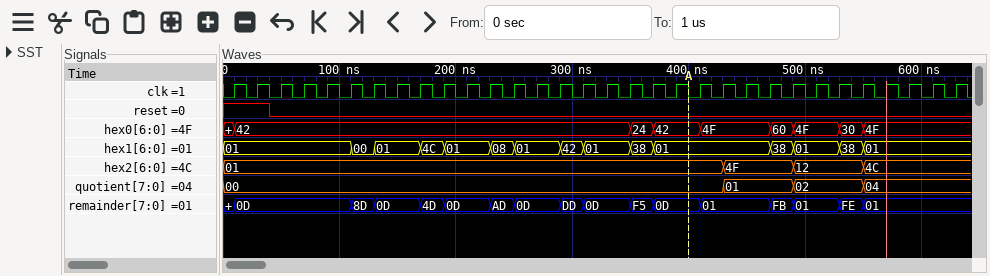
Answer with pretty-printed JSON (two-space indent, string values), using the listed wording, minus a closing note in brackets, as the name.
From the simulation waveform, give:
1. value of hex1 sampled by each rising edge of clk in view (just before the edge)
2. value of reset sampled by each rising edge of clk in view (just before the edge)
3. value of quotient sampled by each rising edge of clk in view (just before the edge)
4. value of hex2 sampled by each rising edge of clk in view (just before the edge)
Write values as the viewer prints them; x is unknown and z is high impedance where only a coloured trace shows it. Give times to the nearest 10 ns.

{
  "value of hex1 sampled by each rising edge of clk in view": "01, 01, 01, 01, 01, 01, 00, 01, 01, 4C, 01, 01, 08, 01, 01, 42, 01, 01, 38, 01, 01, 01, 01, 01, 38, 01, 01, 38, 01, 01, 01, 01",
  "value of reset sampled by each rising edge of clk in view": "1 1 0 0 0 0 0 0 0 0 0 0 0 0 0 0 0 0 0 0 0 0 0 0 0 0 0 0 0 0 0 0",
  "value of quotient sampled by each rising edge of clk in view": "00, 00, 00, 00, 00, 00, 00, 00, 00, 00, 00, 00, 00, 00, 00, 00, 00, 00, 00, 00, 00, 00, 01, 01, 01, 02, 02, 02, 04, 04, 04, 04",
  "value of hex2 sampled by each rising edge of clk in view": "01, 01, 01, 01, 01, 01, 01, 01, 01, 01, 01, 01, 01, 01, 01, 01, 01, 01, 01, 01, 01, 01, 4F, 4F, 4F, 12, 12, 12, 4C, 4C, 4C, 4C"
}
